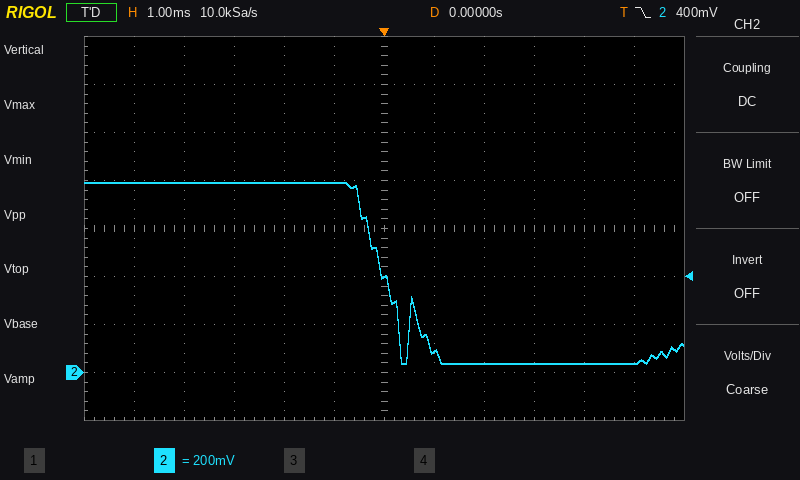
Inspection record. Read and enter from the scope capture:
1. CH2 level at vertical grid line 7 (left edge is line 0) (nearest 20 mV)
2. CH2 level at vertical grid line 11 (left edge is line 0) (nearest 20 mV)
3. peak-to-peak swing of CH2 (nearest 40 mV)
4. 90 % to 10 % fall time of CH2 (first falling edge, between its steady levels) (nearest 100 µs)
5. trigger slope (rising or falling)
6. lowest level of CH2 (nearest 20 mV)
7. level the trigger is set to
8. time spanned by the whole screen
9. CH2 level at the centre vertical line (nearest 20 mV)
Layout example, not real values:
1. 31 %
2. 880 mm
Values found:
1. 80 mV
2. 40 mV
3. 760 mV
4. 800 µs
5. falling
6. 40 mV
7. 400 mV
8. 12 ms
9. 400 mV
